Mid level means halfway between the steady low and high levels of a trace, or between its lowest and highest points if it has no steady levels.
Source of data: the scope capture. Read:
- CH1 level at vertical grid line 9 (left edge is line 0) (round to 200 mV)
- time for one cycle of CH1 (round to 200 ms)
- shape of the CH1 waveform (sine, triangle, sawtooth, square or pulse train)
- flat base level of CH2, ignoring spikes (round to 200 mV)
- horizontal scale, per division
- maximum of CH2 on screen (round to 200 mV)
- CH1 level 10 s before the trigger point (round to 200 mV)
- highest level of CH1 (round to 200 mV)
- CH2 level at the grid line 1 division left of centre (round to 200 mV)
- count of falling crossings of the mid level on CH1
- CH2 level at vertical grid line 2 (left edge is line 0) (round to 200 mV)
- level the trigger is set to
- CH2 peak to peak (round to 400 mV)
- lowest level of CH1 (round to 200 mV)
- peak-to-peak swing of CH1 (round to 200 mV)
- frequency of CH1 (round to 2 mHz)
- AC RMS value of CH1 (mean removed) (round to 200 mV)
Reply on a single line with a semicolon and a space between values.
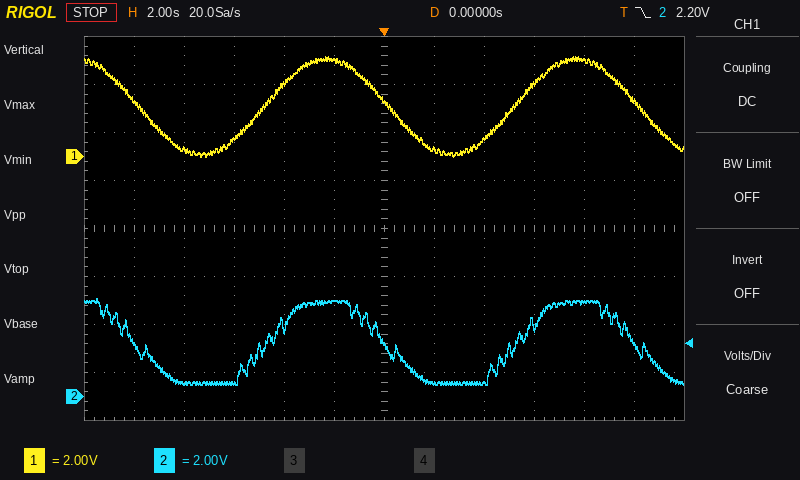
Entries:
3.0 V; 10.0 s; sine; 600 mV; 2 s; 4.0 V; 2.4 V; 4.2 V; 4.0 V; 3; 600 mV; 2.20 V; 3.6 V; 0.0 V; 4.2 V; 100 mHz; 1.4 V
